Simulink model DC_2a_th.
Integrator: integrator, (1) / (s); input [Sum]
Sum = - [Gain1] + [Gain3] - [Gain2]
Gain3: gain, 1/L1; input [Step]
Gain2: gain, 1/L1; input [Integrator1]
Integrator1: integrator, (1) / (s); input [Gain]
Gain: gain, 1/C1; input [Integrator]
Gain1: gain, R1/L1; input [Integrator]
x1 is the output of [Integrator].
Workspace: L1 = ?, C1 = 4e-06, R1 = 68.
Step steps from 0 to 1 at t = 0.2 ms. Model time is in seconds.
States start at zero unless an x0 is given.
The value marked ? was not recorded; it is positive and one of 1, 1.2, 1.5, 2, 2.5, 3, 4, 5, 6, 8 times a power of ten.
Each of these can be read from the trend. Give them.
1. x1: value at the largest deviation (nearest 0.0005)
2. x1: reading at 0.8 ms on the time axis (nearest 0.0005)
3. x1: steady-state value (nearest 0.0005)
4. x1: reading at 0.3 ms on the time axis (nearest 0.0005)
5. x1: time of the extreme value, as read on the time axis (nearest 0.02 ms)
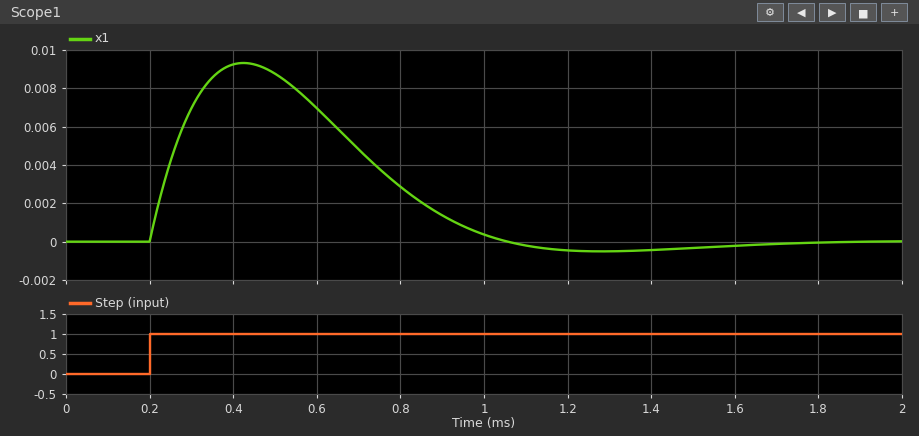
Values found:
0.0095
0.0030
0.0000
0.0070
0.42 ms
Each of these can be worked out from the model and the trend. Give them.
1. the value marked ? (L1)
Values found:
0.01
